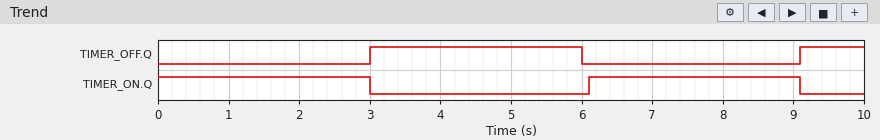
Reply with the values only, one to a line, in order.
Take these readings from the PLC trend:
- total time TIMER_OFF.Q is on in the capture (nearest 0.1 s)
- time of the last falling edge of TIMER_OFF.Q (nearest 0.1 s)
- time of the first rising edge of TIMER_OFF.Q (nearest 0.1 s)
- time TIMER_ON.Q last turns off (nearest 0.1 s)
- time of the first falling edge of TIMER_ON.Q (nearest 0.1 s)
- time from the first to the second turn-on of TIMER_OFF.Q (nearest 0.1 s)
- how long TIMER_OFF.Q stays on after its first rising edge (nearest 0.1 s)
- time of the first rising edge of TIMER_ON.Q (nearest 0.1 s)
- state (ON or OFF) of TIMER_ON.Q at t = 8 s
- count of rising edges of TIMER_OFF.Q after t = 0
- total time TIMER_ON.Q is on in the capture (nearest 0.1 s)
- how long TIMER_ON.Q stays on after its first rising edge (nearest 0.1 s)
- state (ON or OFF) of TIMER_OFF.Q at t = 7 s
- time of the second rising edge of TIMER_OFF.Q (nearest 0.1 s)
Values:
3.9 s
6.0 s
3.0 s
9.1 s
3.0 s
6.1 s
3.0 s
6.1 s
ON
2
6.0 s
3.0 s
OFF
9.1 s
